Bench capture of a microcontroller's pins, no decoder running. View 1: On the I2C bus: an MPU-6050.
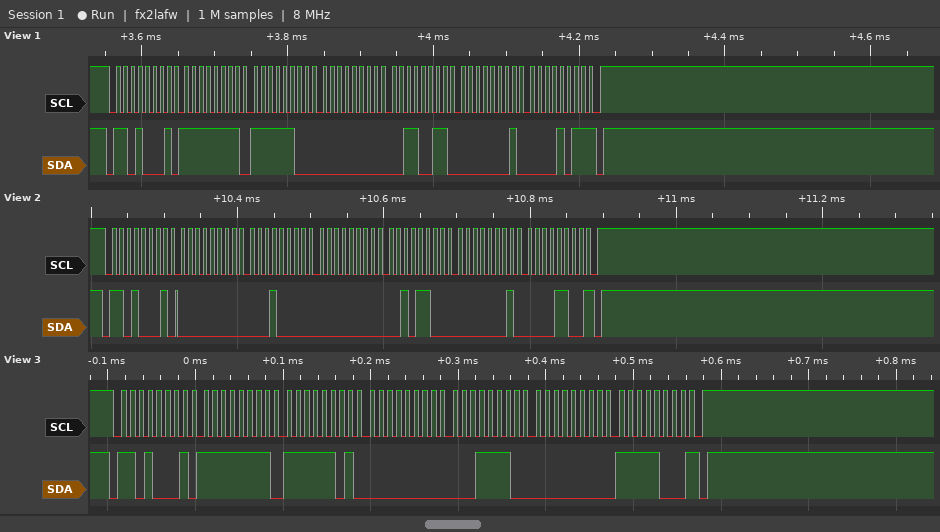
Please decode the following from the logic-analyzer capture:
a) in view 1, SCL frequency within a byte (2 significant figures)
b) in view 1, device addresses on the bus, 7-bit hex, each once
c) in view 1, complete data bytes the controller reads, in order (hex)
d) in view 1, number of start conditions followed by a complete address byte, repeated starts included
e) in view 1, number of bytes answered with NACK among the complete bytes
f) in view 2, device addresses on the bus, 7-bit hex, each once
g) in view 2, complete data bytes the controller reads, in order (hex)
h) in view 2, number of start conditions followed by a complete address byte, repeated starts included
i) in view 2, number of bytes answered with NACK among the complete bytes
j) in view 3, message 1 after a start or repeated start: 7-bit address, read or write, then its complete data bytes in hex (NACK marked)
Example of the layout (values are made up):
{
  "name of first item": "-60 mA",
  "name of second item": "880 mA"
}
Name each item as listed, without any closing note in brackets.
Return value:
{
  "in view 1, SCL frequency within a byte": "100 kHz",
  "in view 1, device addresses on the bus, 7-bit hex, each once": "0x68",
  "in view 1, complete data bytes the controller reads, in order": "FF FC 00 33 01 0B",
  "in view 1, number of start conditions followed by a complete address byte, repeated starts included": "1",
  "in view 1, number of bytes answered with NACK among the complete bytes": "1",
  "in view 2, device addresses on the bus, 7-bit hex, each once": "0x68",
  "in view 2, complete data bytes the controller reads, in order": "00 10 00 2C 01 0C",
  "in view 2, number of start conditions followed by a complete address byte, repeated starts included": "1",
  "in view 2, number of bytes answered with NACK among the complete bytes": "1",
  "in view 3, message 1 after a start or repeated start: 7-bit address, read or write, then its complete data bytes in hex": "0x68 read: FF FD 00 1E 00 F8 NACK"
}
